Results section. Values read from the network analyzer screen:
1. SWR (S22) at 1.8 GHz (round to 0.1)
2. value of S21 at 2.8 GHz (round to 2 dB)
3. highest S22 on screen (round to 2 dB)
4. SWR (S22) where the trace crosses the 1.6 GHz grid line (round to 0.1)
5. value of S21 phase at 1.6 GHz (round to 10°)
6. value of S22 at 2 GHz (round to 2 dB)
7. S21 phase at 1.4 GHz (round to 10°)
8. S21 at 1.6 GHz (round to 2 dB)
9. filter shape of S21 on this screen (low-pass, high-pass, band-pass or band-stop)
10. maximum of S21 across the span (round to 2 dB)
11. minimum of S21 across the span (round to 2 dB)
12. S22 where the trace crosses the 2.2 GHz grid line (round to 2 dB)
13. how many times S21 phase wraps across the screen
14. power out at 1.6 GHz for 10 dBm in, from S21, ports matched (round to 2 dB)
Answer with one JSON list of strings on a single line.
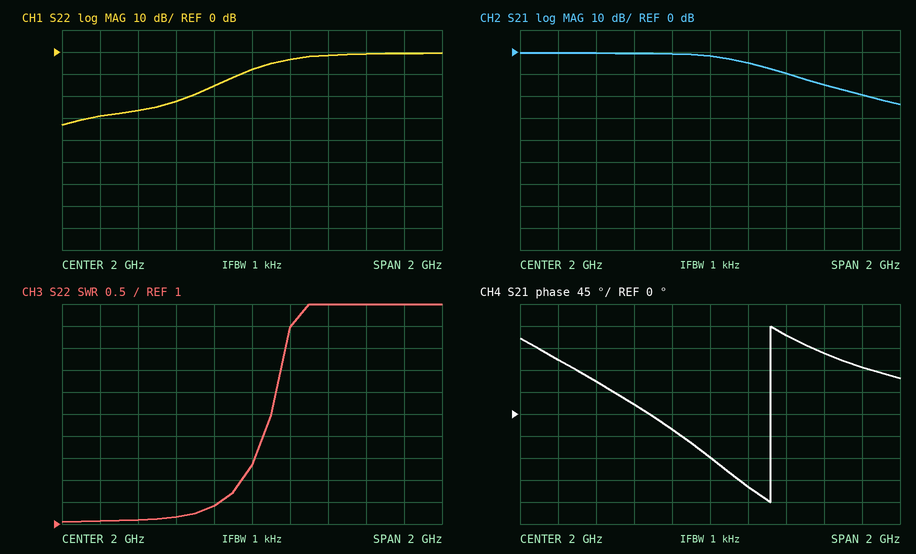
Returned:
["1.4", "-20 dB", "0 dB", "1.2", "20°", "-8 dB", "70°", "0 dB", "low-pass", "0 dB", "-24 dB", "-4 dB", "1", "10 dBm"]
